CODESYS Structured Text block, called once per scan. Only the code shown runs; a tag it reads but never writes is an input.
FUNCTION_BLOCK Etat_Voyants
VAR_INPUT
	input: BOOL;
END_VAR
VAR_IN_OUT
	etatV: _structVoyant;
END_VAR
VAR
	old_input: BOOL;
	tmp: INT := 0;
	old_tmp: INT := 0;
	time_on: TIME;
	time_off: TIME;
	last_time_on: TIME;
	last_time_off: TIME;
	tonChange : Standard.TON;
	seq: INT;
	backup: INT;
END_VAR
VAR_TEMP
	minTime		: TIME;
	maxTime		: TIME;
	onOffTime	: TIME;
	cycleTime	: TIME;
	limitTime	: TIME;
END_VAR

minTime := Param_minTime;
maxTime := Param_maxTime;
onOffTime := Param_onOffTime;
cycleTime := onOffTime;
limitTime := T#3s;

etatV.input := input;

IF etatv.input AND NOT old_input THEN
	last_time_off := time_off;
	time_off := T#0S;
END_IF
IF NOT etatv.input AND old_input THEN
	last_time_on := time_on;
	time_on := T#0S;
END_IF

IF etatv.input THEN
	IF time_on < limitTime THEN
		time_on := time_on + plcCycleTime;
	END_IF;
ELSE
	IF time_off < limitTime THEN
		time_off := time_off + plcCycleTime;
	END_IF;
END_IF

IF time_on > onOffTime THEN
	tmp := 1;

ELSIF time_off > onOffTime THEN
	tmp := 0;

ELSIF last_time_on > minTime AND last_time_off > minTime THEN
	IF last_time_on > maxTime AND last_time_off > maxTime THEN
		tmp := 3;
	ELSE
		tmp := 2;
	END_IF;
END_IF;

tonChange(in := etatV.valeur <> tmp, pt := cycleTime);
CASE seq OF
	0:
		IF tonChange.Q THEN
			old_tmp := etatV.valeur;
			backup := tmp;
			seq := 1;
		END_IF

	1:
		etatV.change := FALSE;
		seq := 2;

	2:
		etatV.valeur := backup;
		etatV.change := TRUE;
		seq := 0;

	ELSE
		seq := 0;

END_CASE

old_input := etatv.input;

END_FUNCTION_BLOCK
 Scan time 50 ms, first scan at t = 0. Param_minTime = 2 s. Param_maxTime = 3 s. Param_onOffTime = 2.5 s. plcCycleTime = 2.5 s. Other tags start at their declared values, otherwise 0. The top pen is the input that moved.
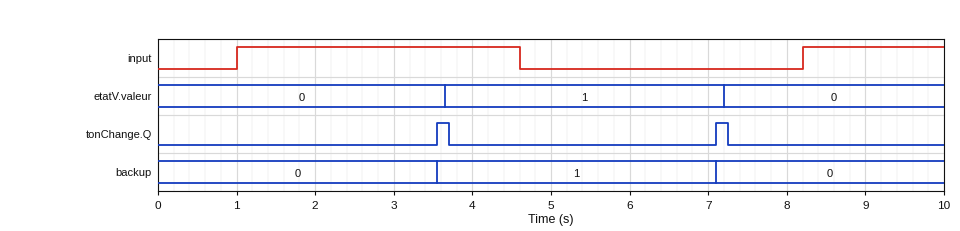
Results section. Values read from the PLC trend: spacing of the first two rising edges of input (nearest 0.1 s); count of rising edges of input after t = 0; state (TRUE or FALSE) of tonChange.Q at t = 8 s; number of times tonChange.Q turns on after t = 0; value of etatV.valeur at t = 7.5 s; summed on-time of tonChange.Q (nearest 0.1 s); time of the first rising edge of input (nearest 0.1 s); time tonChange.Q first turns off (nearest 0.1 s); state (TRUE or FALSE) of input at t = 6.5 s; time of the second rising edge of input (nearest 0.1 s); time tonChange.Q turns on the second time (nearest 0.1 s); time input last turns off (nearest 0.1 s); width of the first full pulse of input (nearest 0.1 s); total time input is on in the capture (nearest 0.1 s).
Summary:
7.2 s
2
FALSE
2
0
0.3 s
1.0 s
3.7 s
FALSE
8.2 s
7.1 s
4.6 s
3.6 s
5.4 s
